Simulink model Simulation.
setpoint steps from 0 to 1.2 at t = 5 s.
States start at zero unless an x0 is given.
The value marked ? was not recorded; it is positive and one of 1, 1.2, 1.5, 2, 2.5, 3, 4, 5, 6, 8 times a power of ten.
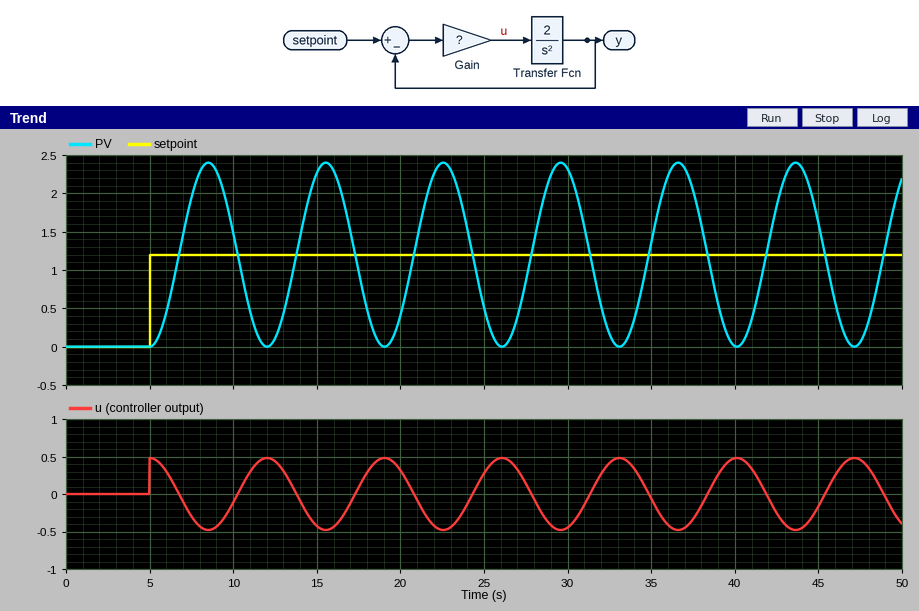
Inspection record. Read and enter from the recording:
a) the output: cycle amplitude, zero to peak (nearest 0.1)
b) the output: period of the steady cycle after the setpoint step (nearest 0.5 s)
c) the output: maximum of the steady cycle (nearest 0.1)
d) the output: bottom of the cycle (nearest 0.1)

1.2
7.0 s
2.4
0.0
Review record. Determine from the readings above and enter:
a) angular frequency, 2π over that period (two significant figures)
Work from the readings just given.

0.90 rad/s
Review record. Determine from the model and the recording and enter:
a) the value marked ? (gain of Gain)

0.4
